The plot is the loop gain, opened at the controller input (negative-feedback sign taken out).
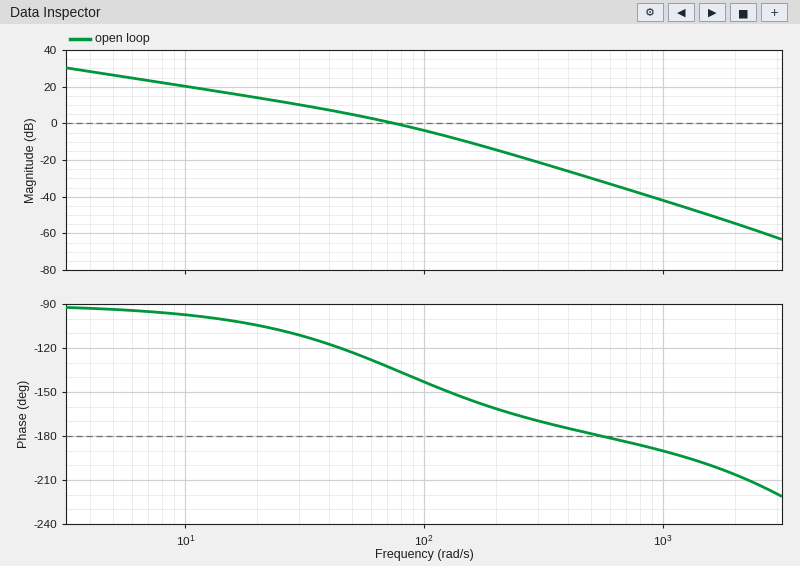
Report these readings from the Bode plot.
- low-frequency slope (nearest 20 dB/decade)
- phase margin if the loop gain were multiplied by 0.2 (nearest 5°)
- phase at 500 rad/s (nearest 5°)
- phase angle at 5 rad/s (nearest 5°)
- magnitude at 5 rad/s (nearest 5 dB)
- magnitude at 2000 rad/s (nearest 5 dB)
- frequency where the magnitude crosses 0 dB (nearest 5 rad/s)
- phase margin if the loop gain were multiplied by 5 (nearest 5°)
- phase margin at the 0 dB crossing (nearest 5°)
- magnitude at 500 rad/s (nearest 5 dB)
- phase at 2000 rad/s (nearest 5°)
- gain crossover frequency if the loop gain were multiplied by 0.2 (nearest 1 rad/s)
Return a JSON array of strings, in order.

["-20 dB/decade", "75°", "-180°", "-95°", "25 dB", "-55 dB", "75 rad/s", "20°", "45°", "-30 dB", "-205°", "20 rad/s"]
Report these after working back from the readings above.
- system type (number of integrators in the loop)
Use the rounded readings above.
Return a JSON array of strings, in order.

["1"]
